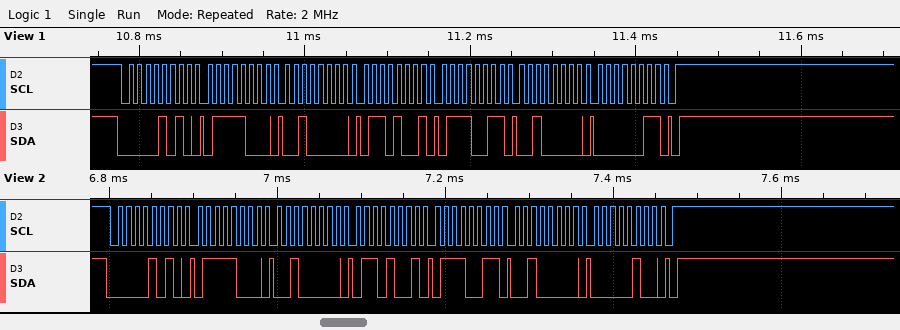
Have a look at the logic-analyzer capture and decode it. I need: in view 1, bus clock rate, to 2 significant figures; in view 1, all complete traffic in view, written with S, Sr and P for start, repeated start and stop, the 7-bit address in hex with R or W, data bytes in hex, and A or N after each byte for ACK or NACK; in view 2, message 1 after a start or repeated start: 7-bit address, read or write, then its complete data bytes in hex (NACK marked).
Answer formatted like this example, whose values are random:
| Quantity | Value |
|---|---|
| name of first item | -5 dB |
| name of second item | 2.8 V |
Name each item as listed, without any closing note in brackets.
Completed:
| Quantity | Value |
|---|---|
| in view 1, bus clock rate, to 2 significant figures | 100 kHz |
| in view 1, all complete traffic in view, written with S, Sr and P for start, repeated start and stop, the 7-bit address in hex with R or W, data bytes in hex, and A or N after each byte for ACK or NACK | S 05W A 78 A 20 A 69 A 73 A 20 A 03 A P |
| in view 2, message 1 after a start or repeated start: 7-bit address, read or write, then its complete data bytes in hex | 0x05 write: 78 20 69 73 20 04 |
